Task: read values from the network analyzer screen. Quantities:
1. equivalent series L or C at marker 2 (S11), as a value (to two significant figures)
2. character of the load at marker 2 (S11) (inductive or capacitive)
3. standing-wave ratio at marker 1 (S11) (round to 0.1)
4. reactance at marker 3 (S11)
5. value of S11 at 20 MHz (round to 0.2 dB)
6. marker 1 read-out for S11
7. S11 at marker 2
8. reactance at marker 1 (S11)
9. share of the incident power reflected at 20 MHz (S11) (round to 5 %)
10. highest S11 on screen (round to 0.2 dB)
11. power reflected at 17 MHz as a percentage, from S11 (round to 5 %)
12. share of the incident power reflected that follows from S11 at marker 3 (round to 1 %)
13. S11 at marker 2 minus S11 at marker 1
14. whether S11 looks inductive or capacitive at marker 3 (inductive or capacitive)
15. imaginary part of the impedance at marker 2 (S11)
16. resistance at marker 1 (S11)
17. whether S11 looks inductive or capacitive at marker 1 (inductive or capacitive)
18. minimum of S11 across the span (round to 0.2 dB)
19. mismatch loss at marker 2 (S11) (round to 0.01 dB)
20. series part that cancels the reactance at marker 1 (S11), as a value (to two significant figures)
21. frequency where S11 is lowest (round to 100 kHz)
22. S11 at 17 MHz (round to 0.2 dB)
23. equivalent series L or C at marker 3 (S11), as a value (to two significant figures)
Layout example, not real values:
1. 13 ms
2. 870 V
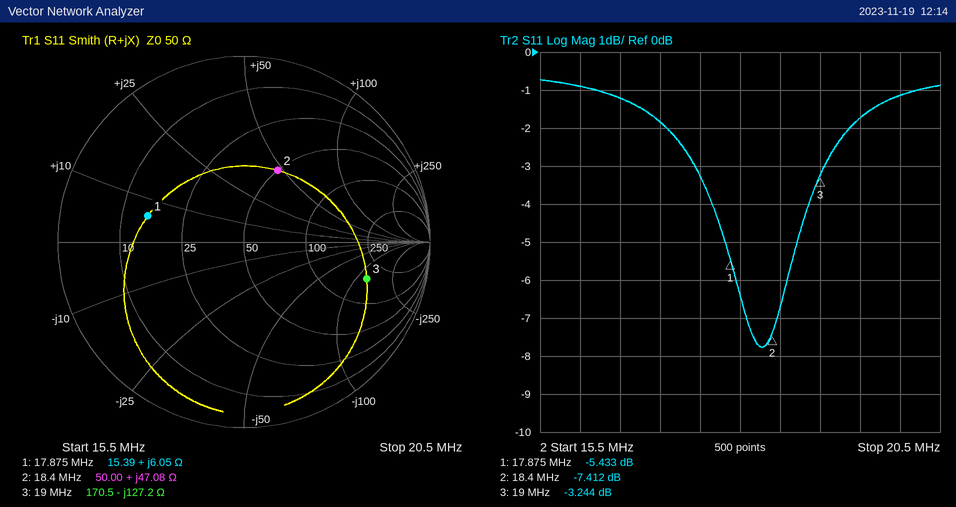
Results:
1. 410 nH
2. inductive
3. 3.3
4. -127.2 Ω
5. -1.2 dB
6. -5.433 dB
7. -7.412 dB
8. +6.05 Ω
9. 75 %
10. -0.8 dB
11. 65 %
12. 47 %
13. -1.979 dB
14. capacitive
15. +47.08 Ω
16. 15.39 Ω
17. inductive
18. -7.8 dB
19. 0.87 dB
20. 1.5 nF
21. 18.3 MHz
22. -1.8 dB
23. 66 pF
